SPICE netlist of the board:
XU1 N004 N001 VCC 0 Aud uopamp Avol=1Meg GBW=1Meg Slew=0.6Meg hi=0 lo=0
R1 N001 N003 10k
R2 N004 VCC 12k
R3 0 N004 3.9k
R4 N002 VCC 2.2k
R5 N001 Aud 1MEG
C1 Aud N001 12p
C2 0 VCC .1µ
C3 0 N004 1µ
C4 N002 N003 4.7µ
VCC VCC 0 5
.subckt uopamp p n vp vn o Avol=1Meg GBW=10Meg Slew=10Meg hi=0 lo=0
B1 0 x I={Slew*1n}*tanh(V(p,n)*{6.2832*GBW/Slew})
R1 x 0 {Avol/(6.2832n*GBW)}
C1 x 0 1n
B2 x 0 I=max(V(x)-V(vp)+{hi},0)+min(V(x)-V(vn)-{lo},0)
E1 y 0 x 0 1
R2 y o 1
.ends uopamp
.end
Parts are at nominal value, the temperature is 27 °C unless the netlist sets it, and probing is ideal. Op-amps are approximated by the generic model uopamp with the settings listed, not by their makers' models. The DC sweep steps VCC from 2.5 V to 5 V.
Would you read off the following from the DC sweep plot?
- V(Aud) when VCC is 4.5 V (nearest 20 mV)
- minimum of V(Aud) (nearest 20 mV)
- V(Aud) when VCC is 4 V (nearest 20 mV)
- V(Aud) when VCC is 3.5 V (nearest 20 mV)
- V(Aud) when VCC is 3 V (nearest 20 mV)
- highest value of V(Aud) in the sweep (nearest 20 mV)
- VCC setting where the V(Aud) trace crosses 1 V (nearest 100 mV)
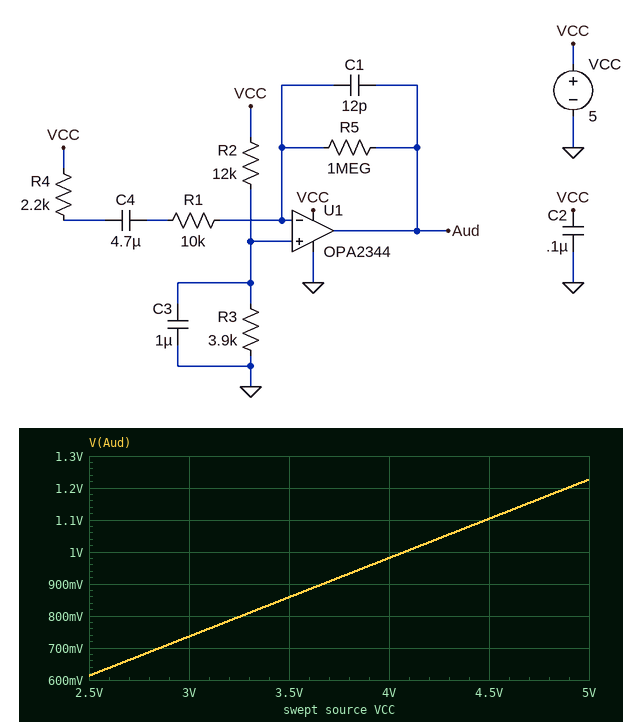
1.10 V
620 mV
980 mV
860 mV
740 mV
1.22 V
4.1 V
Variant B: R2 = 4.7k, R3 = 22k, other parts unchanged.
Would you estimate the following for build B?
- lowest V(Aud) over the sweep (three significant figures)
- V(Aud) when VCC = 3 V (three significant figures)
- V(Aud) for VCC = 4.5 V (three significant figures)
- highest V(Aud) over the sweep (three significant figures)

2.06 V
2.47 V
3.71 V
4.12 V
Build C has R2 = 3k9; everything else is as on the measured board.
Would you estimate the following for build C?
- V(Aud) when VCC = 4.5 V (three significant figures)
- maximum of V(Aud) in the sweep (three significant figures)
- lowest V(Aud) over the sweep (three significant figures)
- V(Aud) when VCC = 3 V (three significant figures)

2.25 V
2.50 V
1.25 V
1.50 V
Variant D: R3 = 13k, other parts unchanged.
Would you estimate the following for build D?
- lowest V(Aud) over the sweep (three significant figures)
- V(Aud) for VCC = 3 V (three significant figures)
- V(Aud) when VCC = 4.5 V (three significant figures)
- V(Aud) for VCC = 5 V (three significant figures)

1.30 V
1.56 V
2.34 V
2.60 V
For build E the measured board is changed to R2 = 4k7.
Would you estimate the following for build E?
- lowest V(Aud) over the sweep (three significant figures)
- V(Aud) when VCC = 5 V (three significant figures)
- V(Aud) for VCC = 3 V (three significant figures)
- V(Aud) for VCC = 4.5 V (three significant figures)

1.13 V
2.27 V
1.36 V
2.04 V
